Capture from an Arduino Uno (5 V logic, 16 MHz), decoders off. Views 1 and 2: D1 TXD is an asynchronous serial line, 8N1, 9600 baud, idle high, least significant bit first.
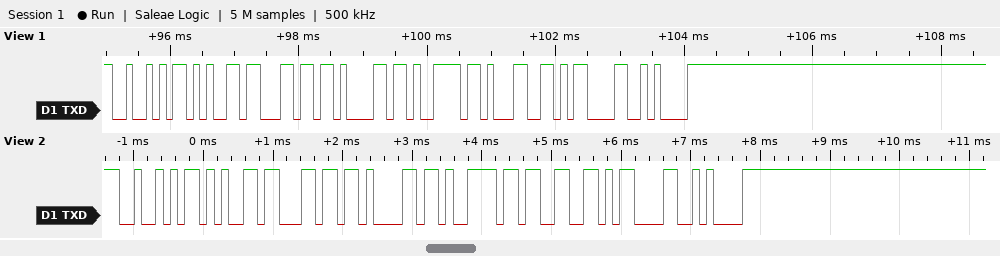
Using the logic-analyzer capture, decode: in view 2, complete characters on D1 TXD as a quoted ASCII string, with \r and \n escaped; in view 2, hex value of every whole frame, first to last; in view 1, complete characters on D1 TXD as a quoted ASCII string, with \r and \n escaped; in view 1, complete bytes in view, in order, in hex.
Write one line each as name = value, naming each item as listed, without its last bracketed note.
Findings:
in view 2, complete characters on D1 TXD as a quoted ASCII string, with \r and \n escaped = "Relay3\r\n"
in view 2, hex value of every whole frame, first to last = 52 65 6C 61 79 33 0D 0A
in view 1, complete characters on D1 TXD as a quoted ASCII string, with \r and \n escaped = "Relay1\r\n"
in view 1, complete bytes in view, in order, in hex = 52 65 6C 61 79 31 0D 0A
